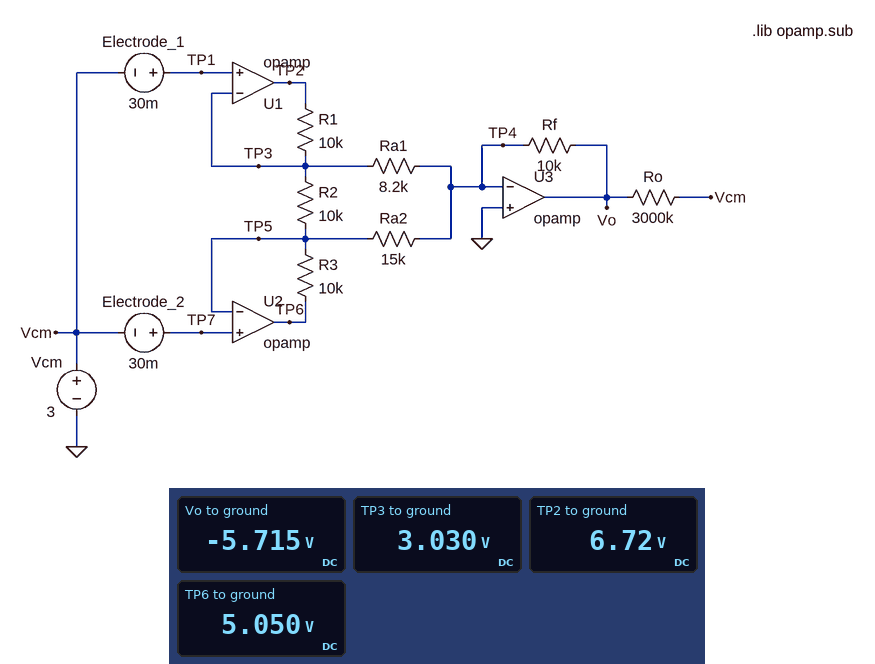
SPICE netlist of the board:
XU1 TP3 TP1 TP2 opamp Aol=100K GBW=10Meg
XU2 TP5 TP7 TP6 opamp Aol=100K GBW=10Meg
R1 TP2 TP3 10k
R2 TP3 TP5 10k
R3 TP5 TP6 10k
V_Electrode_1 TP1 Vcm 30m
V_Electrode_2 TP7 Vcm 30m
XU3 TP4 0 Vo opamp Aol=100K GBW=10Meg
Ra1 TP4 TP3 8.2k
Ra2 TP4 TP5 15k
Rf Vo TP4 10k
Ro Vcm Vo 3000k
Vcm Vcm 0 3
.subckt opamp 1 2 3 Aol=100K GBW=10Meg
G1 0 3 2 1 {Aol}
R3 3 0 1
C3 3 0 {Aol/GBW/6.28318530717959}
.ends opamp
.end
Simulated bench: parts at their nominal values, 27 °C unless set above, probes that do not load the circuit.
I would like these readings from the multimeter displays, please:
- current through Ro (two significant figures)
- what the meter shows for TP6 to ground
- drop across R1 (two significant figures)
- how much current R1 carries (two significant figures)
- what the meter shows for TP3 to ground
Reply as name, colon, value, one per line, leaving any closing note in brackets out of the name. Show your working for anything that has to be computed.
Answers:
current through Ro: (3 V - (-5.715 V)) / 3 MΩ = 2.9 µA
what the meter shows for TP6 to ground: 5.050 V
drop across R1: 6.72 V - 3.03 V = 3.7 V
how much current R1 carries: (6.72 V - 3.03 V) / 10 kΩ = 370 µA
what the meter shows for TP3 to ground: 3.030 V
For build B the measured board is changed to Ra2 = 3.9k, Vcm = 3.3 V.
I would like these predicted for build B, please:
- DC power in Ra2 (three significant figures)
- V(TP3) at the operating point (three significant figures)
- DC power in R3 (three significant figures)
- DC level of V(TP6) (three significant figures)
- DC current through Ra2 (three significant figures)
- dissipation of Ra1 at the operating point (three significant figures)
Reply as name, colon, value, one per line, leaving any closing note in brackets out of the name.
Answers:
DC power in Ra2: 2.84 mW
V(TP3) at the operating point: 3.33 V
DC power in R3: 7.29 mW
DC level of V(TP6): 11.9 V
DC current through Ra2: 854 µA
dissipation of Ra1 at the operating point: 1.35 mW
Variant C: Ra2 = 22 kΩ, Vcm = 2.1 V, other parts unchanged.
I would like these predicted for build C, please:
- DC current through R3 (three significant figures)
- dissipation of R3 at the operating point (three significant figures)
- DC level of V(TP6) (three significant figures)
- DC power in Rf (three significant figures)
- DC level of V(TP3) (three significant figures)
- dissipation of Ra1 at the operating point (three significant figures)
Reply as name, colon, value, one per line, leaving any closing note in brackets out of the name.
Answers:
DC current through R3: 96.8 µA
dissipation of R3 at the operating point: 93.7 µW
DC level of V(TP6): 3.10 V
DC power in Rf: 1.27 mW
DC level of V(TP3): 2.13 V
dissipation of Ra1 at the operating point: 553 µW
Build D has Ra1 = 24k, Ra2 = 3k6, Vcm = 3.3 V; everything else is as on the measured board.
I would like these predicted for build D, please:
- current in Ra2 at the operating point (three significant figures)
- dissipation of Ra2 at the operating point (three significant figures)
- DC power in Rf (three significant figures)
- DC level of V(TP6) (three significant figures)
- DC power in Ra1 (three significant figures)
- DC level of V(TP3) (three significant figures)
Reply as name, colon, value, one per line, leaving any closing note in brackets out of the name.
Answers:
current in Ra2 at the operating point: 925 µA
dissipation of Ra2 at the operating point: 3.08 mW
DC power in Rf: 11.3 mW
DC level of V(TP6): 12.6 V
DC power in Ra1: 462 µW
DC level of V(TP3): 3.33 V
